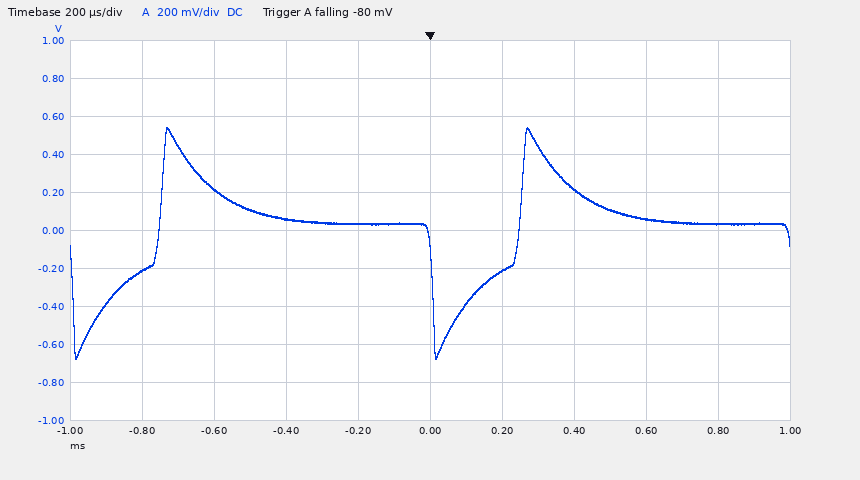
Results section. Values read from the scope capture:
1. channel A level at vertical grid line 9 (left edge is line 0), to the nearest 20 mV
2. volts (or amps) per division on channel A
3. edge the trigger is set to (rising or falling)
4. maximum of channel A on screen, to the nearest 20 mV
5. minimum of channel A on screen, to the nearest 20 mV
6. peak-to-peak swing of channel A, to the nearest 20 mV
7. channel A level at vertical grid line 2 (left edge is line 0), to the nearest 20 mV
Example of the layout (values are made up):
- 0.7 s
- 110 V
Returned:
- 40 mV
- 200 mV
- falling
- 540 mV
- -680 mV
- 1.22 V
- 220 mV
